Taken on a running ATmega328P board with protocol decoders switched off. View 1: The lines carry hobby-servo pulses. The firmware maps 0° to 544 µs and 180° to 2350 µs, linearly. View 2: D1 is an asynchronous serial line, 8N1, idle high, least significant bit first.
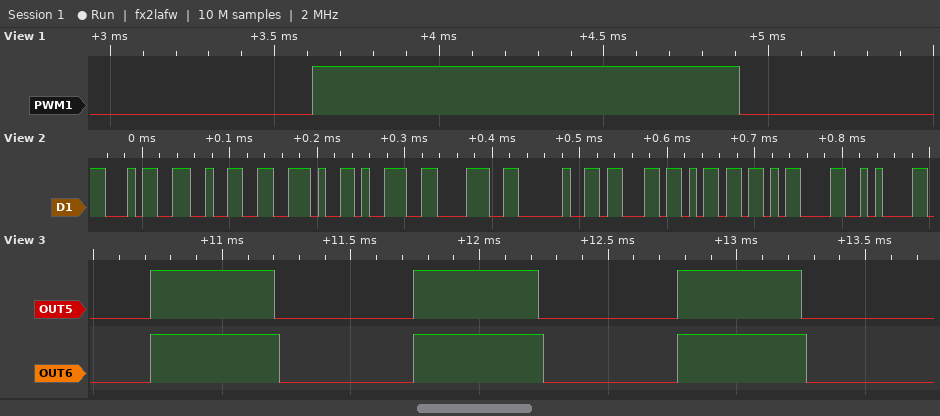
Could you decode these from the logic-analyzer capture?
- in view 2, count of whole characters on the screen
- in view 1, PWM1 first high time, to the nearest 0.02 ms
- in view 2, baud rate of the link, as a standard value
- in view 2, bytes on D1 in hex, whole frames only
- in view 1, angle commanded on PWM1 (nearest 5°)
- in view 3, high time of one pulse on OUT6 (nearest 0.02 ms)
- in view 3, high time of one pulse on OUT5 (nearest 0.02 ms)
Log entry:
10
1.30 ms
115200 baud
34 32 2E 39 38 20 63 6D 0D 0A
75°
0.50 ms
0.48 ms
